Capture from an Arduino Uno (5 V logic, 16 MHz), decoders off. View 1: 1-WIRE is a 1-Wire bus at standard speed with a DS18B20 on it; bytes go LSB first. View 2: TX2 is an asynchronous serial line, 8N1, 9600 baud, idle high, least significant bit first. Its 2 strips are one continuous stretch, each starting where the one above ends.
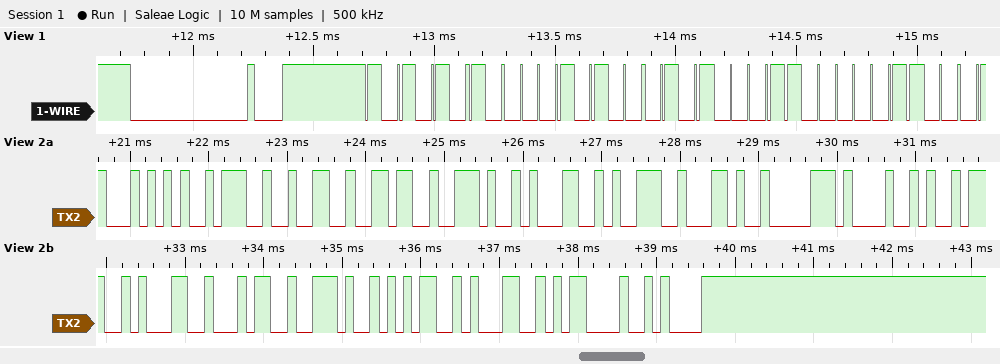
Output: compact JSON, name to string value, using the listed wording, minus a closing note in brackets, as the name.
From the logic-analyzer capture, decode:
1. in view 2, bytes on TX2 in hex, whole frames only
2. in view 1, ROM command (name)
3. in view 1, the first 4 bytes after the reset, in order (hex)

{"in view 2, bytes on TX2 in hex, whole frames only": "54 3A 32 36 2E 31 39 2C 70 48 3A 31 34 2E 35 31 0D 0A", "in view 1, ROM command": "Match ROM", "in view 1, the first 4 bytes after the reset, in order": "55 28 8A C1"}
